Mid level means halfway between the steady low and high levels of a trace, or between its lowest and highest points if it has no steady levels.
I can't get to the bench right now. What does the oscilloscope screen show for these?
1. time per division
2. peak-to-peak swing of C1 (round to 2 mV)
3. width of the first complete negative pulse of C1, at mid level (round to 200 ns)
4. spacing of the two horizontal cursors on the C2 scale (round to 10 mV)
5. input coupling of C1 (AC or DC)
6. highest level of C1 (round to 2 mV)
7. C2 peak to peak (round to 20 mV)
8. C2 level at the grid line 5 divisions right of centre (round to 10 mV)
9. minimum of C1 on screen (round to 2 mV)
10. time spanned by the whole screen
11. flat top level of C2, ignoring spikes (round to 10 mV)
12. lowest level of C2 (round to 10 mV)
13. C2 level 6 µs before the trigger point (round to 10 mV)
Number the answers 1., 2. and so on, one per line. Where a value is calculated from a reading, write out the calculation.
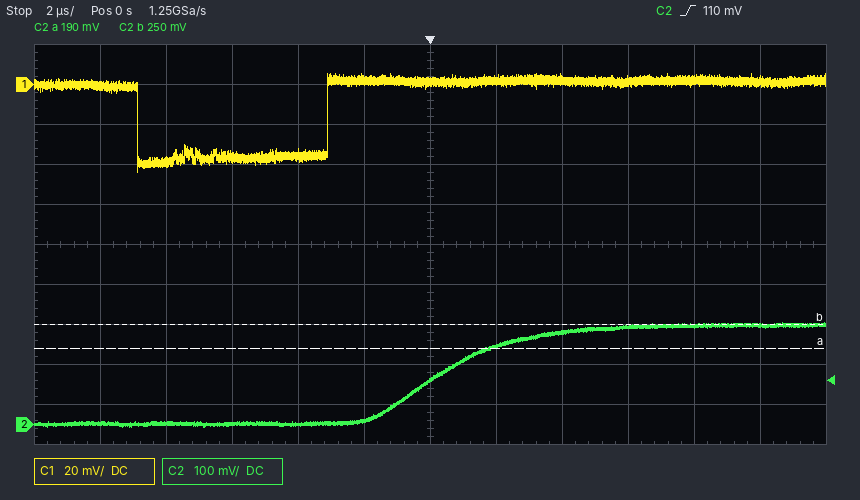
1. 2 µs
2. 6 mV − (-44 mV) = 50 mV
3. 5.8 µs
4. 60 mV
5. DC
6. 6 mV
7. 260 mV
8. 250 mV
9. -44 mV
10. 24 µs
11. 250 mV
12. -10 mV
13. 0 mV
